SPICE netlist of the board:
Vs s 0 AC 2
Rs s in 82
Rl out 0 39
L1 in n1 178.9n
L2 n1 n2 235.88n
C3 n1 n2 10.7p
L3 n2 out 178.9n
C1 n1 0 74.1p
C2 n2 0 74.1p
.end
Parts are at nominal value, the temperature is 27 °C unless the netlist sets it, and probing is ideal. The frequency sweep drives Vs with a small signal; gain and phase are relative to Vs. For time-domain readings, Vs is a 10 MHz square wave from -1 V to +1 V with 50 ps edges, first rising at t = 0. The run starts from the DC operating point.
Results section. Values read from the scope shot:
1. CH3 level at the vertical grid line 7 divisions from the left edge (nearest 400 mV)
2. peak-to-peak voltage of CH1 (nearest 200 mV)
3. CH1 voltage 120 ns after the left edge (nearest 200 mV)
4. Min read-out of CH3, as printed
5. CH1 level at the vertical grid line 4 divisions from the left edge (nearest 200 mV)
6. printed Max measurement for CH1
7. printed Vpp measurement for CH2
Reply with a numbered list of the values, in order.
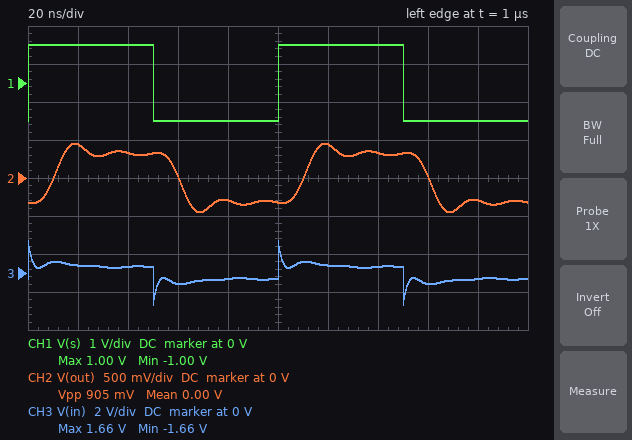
1. 400 mV
2. 2.0 V
3. 1.0 V
4. -1.66 V
5. -1.0 V
6. 1.00 V
7. 905 mV
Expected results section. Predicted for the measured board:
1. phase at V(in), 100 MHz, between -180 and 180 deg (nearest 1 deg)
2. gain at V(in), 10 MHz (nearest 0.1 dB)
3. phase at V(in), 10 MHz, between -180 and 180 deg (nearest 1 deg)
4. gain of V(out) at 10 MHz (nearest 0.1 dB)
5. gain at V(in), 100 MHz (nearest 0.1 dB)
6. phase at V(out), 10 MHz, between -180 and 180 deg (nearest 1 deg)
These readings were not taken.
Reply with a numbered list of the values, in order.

1. 42 deg
2. -8.0 dB
3. 15 deg
4. -9.7 dB
5. -2.6 dB
6. -32 deg
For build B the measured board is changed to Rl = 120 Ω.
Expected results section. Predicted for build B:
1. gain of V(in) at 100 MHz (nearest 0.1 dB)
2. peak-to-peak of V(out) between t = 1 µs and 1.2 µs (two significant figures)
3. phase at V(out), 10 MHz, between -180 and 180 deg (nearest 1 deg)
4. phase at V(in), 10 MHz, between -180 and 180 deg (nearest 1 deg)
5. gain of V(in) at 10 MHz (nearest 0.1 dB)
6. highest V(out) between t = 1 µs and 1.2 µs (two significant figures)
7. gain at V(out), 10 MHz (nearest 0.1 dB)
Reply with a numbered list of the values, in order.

1. -2.6 dB
2. 1.4 V
3. -36 deg
4. -17 deg
5. -5.9 dB
6. 710 mV
7. -4.8 dB
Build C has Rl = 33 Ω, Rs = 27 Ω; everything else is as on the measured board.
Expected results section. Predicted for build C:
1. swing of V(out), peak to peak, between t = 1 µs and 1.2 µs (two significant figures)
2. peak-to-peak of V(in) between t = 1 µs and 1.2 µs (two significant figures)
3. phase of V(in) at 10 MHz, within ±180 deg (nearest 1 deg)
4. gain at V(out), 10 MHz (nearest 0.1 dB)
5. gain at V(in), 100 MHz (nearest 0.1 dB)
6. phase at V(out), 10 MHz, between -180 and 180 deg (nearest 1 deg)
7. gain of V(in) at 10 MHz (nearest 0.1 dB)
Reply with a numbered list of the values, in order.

1. 1.2 V
2. 2.9 V
3. 11 deg
4. -6.0 dB
5. -0.4 dB
6. -41 deg
7. -3.4 dB
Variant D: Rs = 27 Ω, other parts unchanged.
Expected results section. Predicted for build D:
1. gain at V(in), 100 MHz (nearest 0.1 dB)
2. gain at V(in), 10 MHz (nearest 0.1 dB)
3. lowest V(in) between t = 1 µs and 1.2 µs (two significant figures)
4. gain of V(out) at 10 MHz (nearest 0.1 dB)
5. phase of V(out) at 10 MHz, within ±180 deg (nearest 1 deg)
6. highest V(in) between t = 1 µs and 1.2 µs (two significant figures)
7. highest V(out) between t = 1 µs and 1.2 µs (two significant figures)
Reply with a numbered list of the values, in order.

1. -0.4 dB
2. -3.4 dB
3. -1.4 V
4. -5.1 dB
5. -39 deg
6. 1.4 V
7. 700 mV
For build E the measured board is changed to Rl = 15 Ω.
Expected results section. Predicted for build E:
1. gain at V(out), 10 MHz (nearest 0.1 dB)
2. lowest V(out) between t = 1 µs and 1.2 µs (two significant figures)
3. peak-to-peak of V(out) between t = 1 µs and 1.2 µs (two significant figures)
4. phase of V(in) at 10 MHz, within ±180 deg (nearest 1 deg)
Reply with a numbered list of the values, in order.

1. -15.8 dB
2. -240 mV
3. 480 mV
4. 41 deg
